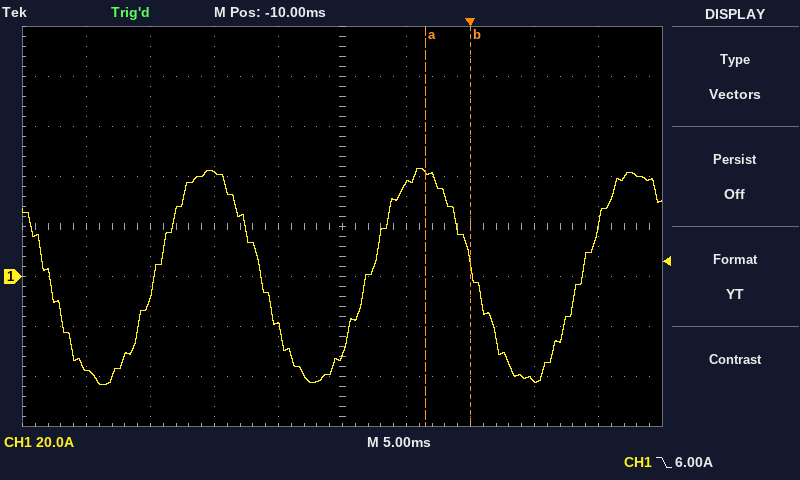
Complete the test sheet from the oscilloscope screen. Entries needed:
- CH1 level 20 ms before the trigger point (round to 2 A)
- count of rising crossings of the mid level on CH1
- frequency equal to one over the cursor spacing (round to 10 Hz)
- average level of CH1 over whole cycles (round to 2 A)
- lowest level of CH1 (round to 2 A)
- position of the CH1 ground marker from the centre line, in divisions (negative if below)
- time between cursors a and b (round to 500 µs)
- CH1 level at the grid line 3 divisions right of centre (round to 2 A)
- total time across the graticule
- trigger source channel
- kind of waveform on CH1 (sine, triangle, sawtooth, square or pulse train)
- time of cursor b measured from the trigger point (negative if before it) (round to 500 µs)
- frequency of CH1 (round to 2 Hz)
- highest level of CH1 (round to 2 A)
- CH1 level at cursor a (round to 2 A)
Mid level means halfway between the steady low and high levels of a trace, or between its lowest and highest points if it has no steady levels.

42 A
3
290 Hz
0 A
-44 A
-1.0 div
3.5 ms
-42 A
50 ms
CH1
sine
0.0 ms
60 Hz
44 A
42 A
